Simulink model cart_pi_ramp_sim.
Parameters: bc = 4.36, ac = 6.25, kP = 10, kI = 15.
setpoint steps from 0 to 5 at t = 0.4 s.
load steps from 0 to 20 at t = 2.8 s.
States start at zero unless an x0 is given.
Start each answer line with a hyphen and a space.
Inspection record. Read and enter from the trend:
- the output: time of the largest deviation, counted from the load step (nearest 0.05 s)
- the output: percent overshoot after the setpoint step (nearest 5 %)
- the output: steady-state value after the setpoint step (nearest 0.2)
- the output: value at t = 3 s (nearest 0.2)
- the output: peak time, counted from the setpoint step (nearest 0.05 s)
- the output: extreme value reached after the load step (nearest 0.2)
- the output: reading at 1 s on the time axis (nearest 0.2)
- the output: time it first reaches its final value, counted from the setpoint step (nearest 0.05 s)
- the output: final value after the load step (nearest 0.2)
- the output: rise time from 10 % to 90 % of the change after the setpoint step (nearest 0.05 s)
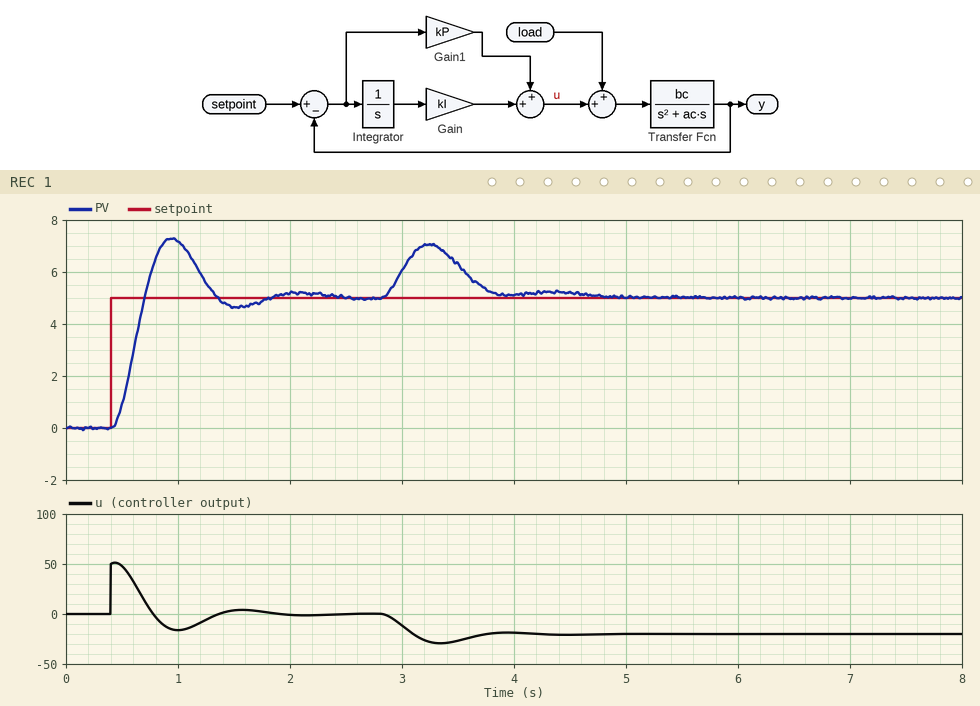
- 0.45 s
- 45 %
- 5.0
- 6.0
- 0.55 s
- 7.0
- 7.2
- 0.30 s
- 5.0
- 0.20 s
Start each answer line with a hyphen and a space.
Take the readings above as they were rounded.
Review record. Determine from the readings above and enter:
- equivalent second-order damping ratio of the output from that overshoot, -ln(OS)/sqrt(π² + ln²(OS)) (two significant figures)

- 0.25
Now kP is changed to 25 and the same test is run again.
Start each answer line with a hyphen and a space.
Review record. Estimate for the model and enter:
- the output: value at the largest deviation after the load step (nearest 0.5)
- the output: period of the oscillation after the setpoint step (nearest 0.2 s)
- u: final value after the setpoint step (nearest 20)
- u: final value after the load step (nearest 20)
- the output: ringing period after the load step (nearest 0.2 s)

- 6.0
- 0.6 s
- 0
- -20
- 0.6 s
